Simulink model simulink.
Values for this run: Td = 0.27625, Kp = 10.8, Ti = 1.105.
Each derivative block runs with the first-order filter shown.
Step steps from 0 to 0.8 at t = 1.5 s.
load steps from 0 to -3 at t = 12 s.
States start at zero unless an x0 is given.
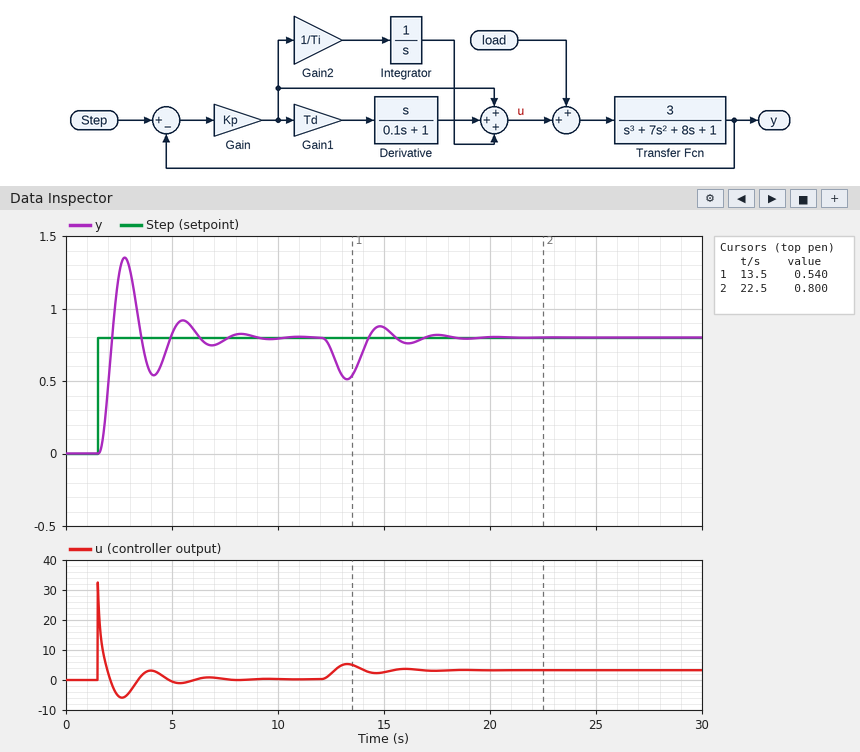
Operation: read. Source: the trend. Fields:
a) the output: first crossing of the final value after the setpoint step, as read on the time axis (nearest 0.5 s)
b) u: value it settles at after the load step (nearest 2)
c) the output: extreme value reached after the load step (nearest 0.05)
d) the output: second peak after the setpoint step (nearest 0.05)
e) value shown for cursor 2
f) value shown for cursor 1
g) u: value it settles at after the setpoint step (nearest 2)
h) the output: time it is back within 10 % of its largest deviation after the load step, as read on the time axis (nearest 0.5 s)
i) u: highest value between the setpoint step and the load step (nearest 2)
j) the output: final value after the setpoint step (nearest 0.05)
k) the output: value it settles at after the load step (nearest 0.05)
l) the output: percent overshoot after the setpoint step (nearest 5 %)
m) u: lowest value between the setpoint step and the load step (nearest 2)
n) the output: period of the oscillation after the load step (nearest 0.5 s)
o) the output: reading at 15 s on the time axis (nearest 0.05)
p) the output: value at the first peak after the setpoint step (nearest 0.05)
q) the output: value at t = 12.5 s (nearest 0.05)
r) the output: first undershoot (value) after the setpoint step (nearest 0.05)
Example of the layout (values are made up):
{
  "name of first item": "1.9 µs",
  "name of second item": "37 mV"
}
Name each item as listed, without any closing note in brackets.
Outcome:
{
  "the output: first crossing of the final value after the setpoint step, as read on the time axis": "2.0 s",
  "u: value it settles at after the load step": "4",
  "the output: extreme value reached after the load step": "0.50",
  "the output: second peak after the setpoint step": "0.90",
  "value shown for cursor 2": "0.800",
  "value shown for cursor 1": "0.540",
  "u: value it settles at after the setpoint step": "0",
  "the output: time it is back within 10 % of its largest deviation after the load step, as read on the time axis": "16.5 s",
  "u: highest value between the setpoint step and the load step": "32",
  "the output: final value after the setpoint step": "0.80",
  "the output: value it settles at after the load step": "0.80",
  "the output: percent overshoot after the setpoint step": "70 %",
  "u: lowest value between the setpoint step and the load step": "-6",
  "the output: period of the oscillation after the load step": "3.0 s",
  "the output: reading at 15 s on the time axis": "0.85",
  "the output: value at the first peak after the setpoint step": "1.35",
  "the output: value at t = 12.5 s": "0.70",
  "the output: first undershoot (value) after the setpoint step": "0.55"
}
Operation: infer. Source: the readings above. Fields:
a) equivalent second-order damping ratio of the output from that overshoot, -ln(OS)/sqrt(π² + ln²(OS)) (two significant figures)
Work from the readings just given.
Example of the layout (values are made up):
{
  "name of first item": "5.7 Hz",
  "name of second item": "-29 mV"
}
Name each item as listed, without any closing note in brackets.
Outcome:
{
  "equivalent second-order damping ratio of the output from that overshoot, -ln(OS)/sqrt(π² + ln²(OS))": "0.11"
}
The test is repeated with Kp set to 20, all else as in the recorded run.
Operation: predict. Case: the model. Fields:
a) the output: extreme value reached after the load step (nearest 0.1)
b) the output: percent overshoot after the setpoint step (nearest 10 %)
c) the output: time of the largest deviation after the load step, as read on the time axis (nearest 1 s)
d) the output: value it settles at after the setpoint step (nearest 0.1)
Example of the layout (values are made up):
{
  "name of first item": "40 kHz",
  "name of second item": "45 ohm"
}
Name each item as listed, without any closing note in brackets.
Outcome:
{
  "the output: extreme value reached after the load step": "0.6",
  "the output: percent overshoot after the setpoint step": "80 %",
  "the output: time of the largest deviation after the load step, as read on the time axis": "13 s",
  "the output: value it settles at after the setpoint step": "0.8"
}
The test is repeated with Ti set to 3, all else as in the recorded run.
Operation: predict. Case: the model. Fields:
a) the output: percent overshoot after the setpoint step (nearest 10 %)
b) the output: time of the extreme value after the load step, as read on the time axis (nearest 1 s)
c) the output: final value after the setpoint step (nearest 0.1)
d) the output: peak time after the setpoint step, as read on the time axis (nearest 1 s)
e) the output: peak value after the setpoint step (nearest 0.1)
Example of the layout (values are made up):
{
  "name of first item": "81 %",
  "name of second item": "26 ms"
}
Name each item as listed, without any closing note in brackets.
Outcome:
{
  "the output: percent overshoot after the setpoint step": "50 %",
  "the output: time of the extreme value after the load step, as read on the time axis": "13 s",
  "the output: final value after the setpoint step": "0.8",
  "the output: peak time after the setpoint step, as read on the time axis": "3 s",
  "the output: peak value after the setpoint step": "1.2"
}
